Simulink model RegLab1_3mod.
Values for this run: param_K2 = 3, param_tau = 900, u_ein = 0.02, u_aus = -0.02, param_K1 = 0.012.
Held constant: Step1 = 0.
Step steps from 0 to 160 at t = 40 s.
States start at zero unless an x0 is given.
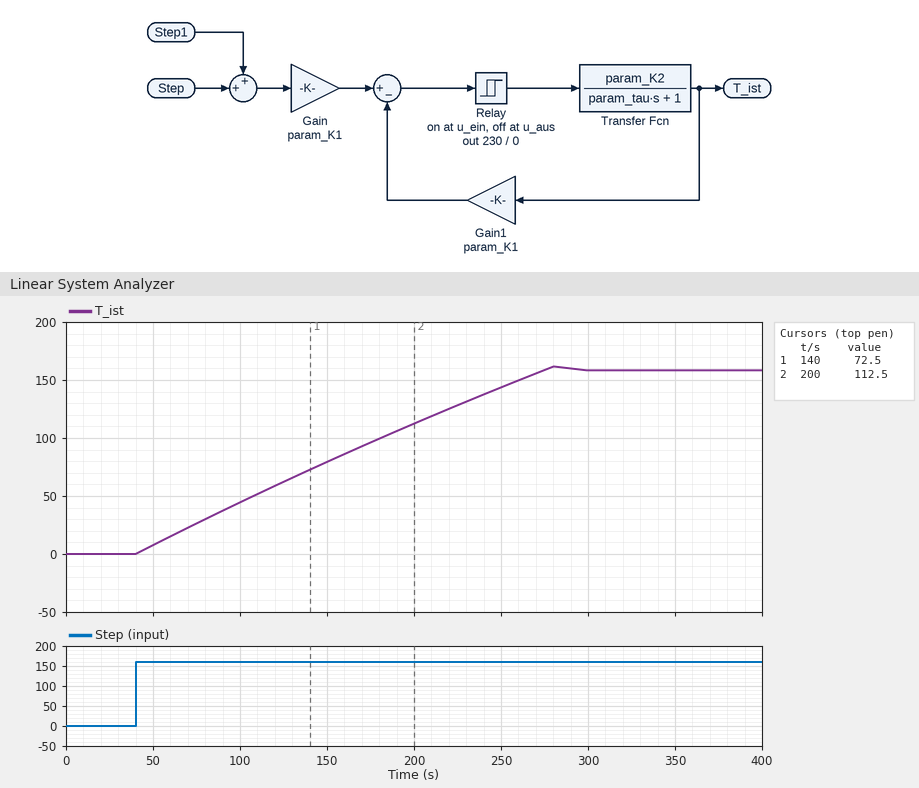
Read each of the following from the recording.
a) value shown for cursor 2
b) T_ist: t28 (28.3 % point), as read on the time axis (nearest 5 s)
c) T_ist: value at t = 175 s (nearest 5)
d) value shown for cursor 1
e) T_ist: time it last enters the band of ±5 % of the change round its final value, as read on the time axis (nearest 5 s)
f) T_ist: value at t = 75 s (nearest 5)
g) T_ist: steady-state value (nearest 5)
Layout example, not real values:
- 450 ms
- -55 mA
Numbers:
- 112.5
- 100 s
- 95
- 72.5
- 260 s
- 25
- 160
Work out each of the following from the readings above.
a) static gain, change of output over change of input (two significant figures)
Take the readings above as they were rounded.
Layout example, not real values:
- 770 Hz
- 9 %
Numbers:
- 1.0
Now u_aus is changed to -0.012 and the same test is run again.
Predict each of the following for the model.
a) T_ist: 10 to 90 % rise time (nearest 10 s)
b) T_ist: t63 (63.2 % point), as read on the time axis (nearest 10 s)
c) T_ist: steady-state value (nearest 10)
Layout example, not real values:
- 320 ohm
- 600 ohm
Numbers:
- 190 s
- 180 s
- 160
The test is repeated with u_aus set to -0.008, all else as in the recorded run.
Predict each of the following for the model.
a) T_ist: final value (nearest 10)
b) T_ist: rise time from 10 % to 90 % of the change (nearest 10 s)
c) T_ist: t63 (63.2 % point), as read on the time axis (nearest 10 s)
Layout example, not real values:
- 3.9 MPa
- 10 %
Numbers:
- 160
- 190 s
- 180 s
